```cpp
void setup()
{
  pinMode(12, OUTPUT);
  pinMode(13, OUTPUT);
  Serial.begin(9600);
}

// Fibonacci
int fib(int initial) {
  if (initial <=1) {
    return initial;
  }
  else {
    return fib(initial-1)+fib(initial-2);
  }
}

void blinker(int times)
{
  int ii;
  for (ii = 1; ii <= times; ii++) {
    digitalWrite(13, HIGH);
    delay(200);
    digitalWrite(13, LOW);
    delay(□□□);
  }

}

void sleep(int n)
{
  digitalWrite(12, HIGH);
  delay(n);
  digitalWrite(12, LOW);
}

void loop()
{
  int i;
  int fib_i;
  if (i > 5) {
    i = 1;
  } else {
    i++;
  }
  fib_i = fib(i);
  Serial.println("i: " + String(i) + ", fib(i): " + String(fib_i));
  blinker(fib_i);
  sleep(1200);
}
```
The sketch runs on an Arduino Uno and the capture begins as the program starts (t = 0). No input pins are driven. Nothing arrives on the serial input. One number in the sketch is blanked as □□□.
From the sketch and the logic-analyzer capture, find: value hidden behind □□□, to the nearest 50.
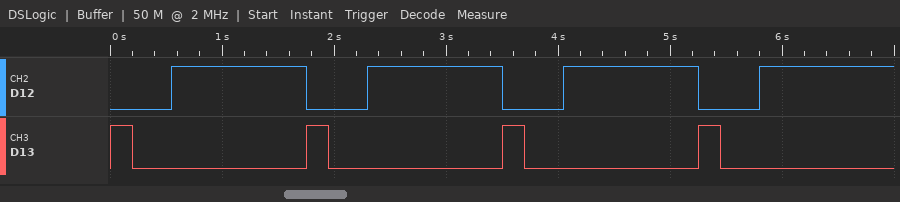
350
